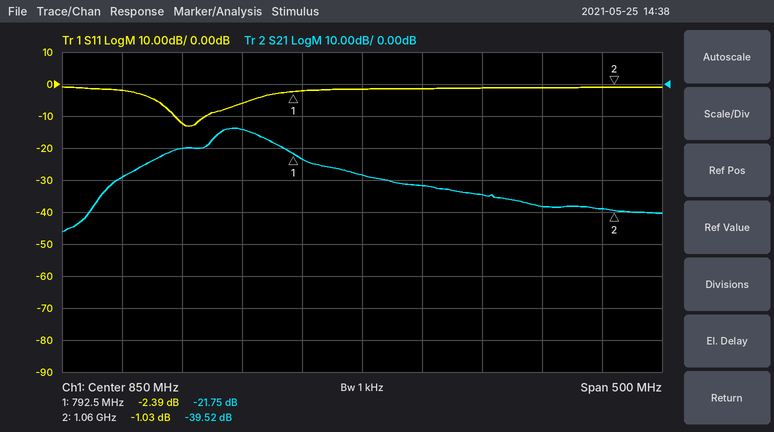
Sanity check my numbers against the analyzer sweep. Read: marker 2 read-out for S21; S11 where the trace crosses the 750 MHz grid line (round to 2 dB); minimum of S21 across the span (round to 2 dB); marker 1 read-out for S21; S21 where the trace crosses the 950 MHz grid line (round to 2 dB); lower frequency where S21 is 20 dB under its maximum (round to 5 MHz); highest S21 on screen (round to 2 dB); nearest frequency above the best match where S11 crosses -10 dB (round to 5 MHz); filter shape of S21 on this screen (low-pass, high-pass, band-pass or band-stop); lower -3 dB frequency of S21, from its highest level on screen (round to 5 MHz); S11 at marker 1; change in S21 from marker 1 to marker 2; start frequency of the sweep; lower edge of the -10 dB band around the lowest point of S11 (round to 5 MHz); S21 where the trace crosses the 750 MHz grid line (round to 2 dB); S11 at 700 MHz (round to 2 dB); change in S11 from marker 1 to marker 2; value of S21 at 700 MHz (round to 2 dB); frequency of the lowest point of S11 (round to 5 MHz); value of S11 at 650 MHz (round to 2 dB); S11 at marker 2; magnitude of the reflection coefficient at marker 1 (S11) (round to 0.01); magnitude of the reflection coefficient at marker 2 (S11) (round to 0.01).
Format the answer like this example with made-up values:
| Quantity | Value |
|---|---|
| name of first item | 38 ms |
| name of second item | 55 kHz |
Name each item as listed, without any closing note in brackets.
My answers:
| Quantity | Value |
|---|---|
| marker 2 read-out for S21 | -39.52 dB |
| S11 where the trace crosses the 750 MHz grid line | -6 dB |
| minimum of S21 across the span | -46 dB |
| marker 1 read-out for S21 | -21.75 dB |
| S21 where the trace crosses the 950 MHz grid line | -34 dB |
| lower frequency where S21 is 20 dB under its maximum | 635 MHz |
| highest S21 on screen | -14 dB |
| nearest frequency above the best match where S11 crosses -10 dB | 720 MHz |
| filter shape of S21 on this screen | band-pass |
| lower -3 dB frequency of S21, from its highest level on screen | 725 MHz |
| S11 at marker 1 | -2.39 dB |
| change in S21 from marker 1 to marker 2 | -17.77 dB |
| start frequency of the sweep | 600 MHz |
| lower edge of the -10 dB band around the lowest point of S11 | 695 MHz |
| S21 where the trace crosses the 750 MHz grid line | -14 dB |
| S11 at 700 MHz | -12 dB |
| change in S11 from marker 1 to marker 2 | 1.36 dB |
| value of S21 at 700 MHz | -20 dB |
| frequency of the lowest point of S11 | 705 MHz |
| value of S11 at 650 MHz | -2 dB |
| S11 at marker 2 | -1.03 dB |
| magnitude of the reflection coefficient at marker 1 (S11) | 0.76 |
| magnitude of the reflection coefficient at marker 2 (S11) | 0.89 |
